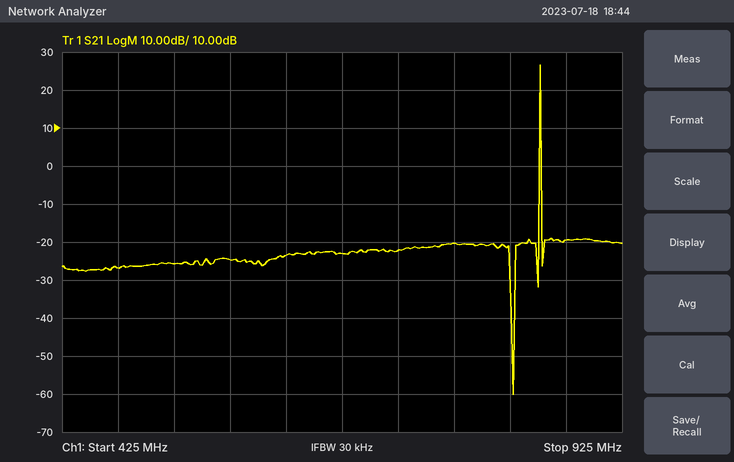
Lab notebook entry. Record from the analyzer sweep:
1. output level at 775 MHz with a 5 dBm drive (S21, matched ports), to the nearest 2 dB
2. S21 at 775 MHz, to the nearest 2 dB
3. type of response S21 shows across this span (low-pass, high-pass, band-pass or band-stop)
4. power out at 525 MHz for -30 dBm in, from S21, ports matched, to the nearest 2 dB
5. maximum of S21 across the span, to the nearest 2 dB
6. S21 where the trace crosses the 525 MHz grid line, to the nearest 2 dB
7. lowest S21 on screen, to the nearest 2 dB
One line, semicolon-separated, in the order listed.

-16 dBm; -20 dB; band-pass; -56 dBm; 26 dB; -26 dB; -60 dB
